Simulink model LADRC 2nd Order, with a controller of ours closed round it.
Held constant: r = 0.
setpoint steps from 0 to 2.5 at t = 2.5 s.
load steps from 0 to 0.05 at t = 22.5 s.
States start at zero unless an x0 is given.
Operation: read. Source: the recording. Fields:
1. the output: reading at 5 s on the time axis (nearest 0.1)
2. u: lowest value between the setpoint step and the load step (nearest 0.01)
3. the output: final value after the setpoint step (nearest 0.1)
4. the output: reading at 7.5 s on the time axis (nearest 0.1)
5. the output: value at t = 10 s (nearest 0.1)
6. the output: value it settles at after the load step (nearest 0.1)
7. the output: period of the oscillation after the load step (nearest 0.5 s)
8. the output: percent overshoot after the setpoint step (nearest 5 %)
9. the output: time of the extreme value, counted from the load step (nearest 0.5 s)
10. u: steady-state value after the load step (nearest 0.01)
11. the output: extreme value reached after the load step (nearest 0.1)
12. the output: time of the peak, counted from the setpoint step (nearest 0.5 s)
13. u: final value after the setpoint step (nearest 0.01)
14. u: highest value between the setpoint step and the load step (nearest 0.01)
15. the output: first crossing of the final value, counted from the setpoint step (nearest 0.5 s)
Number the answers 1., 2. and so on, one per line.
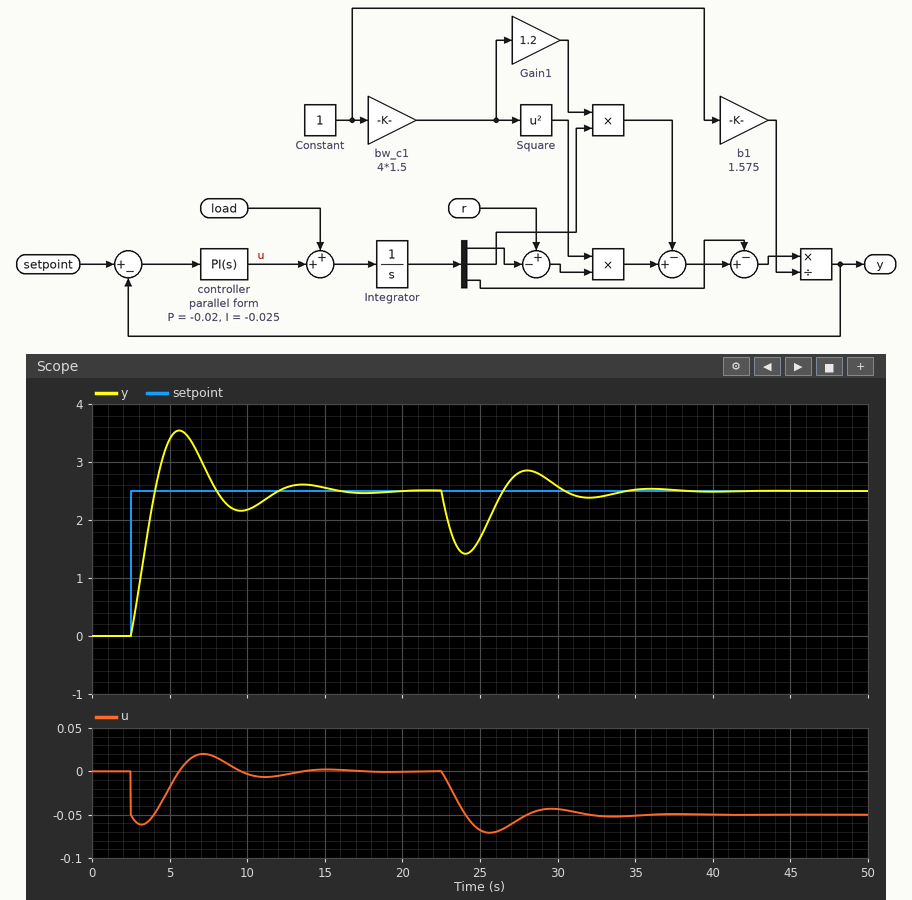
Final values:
1. 3.4
2. -0.06
3. 2.5
4. 2.8
5. 2.2
6. 2.5
7. 8.0 s
8. 40 %
9. 1.5 s
10. -0.05
11. 1.4
12. 3.0 s
13. 0.00
14. 0.02
15. 1.5 s
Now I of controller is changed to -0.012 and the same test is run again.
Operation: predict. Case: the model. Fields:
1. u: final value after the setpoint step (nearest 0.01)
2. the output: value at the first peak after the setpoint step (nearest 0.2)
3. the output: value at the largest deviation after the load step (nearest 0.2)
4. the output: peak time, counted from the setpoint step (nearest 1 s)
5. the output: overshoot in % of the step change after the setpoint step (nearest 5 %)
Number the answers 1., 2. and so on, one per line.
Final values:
1. 0.00
2. 3.2
3. 1.2
4. 4 s
5. 30 %
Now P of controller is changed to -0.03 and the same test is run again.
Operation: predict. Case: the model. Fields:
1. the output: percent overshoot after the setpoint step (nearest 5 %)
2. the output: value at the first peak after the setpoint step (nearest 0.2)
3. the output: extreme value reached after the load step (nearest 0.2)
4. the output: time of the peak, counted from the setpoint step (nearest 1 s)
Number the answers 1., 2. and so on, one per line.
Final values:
1. 30 %
2. 3.2
3. 1.6
4. 3 s
